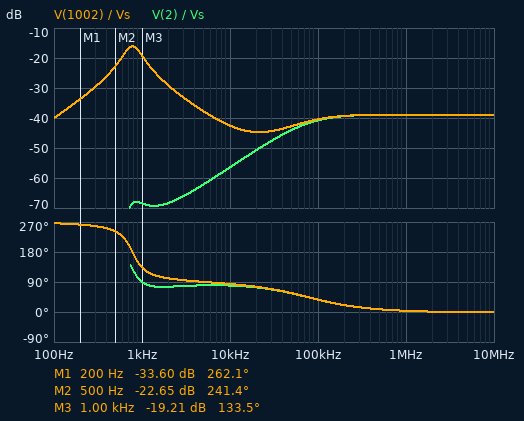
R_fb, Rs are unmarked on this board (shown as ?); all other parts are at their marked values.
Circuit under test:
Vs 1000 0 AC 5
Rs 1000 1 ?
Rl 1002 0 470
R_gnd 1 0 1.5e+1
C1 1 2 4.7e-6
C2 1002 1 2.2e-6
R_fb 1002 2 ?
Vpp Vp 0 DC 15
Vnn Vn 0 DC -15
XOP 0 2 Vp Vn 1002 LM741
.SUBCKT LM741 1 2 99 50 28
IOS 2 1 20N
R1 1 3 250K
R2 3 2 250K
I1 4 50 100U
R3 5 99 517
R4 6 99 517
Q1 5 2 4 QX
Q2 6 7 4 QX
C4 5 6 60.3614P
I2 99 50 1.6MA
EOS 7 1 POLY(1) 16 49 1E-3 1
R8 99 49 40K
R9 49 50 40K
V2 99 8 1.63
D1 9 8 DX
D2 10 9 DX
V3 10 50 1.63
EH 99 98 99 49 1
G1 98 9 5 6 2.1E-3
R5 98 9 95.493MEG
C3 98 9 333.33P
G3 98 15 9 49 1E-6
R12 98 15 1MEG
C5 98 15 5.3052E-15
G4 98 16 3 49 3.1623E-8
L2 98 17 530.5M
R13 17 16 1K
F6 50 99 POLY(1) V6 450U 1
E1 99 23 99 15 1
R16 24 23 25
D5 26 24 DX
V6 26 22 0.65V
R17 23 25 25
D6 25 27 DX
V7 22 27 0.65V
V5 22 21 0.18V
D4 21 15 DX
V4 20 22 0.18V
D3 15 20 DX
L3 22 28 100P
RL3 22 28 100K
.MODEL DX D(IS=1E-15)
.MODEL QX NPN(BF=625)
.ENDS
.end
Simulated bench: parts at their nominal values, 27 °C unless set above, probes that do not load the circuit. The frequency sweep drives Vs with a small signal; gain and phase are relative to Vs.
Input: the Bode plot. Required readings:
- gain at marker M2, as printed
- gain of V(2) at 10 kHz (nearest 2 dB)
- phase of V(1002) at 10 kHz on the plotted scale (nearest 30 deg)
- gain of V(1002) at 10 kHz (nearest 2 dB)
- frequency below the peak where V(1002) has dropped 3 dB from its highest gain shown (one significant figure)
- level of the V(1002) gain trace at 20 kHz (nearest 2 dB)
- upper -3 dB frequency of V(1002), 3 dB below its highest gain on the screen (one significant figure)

-22.65 dB
-56 dB
90 deg
-42 dB
600 Hz
-44 dB
1 kHz
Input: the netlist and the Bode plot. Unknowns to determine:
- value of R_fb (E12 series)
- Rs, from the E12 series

270 Ω
1.2 kΩ
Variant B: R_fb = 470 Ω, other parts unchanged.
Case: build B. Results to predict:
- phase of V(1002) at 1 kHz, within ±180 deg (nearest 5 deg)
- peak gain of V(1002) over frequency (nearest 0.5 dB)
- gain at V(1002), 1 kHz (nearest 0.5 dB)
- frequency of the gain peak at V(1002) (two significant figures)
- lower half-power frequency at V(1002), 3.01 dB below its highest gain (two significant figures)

110 deg
-11.5 dB
-21.0 dB
590 Hz
490 Hz
